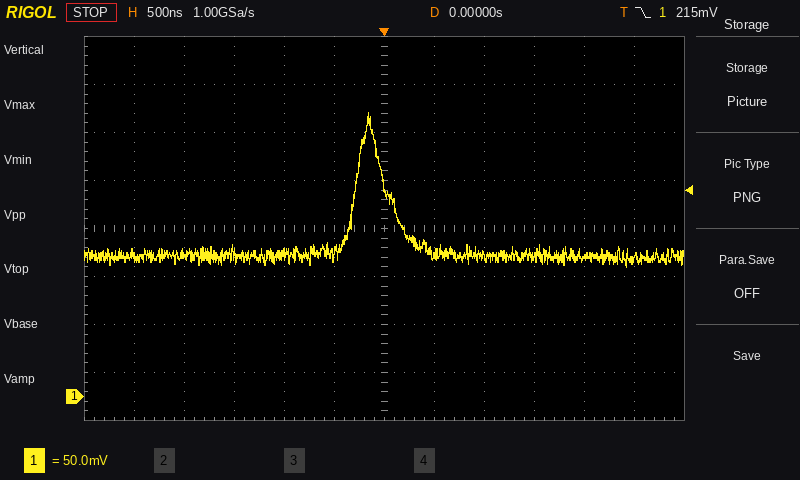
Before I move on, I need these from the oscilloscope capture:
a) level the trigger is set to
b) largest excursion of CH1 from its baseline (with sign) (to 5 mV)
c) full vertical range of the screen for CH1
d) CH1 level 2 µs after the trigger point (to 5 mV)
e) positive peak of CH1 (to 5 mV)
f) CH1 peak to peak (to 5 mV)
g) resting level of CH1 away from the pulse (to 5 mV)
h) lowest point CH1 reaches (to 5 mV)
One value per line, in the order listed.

215 mV
+150 mV
400 mV
145 mV
295 mV
160 mV
145 mV
135 mV
